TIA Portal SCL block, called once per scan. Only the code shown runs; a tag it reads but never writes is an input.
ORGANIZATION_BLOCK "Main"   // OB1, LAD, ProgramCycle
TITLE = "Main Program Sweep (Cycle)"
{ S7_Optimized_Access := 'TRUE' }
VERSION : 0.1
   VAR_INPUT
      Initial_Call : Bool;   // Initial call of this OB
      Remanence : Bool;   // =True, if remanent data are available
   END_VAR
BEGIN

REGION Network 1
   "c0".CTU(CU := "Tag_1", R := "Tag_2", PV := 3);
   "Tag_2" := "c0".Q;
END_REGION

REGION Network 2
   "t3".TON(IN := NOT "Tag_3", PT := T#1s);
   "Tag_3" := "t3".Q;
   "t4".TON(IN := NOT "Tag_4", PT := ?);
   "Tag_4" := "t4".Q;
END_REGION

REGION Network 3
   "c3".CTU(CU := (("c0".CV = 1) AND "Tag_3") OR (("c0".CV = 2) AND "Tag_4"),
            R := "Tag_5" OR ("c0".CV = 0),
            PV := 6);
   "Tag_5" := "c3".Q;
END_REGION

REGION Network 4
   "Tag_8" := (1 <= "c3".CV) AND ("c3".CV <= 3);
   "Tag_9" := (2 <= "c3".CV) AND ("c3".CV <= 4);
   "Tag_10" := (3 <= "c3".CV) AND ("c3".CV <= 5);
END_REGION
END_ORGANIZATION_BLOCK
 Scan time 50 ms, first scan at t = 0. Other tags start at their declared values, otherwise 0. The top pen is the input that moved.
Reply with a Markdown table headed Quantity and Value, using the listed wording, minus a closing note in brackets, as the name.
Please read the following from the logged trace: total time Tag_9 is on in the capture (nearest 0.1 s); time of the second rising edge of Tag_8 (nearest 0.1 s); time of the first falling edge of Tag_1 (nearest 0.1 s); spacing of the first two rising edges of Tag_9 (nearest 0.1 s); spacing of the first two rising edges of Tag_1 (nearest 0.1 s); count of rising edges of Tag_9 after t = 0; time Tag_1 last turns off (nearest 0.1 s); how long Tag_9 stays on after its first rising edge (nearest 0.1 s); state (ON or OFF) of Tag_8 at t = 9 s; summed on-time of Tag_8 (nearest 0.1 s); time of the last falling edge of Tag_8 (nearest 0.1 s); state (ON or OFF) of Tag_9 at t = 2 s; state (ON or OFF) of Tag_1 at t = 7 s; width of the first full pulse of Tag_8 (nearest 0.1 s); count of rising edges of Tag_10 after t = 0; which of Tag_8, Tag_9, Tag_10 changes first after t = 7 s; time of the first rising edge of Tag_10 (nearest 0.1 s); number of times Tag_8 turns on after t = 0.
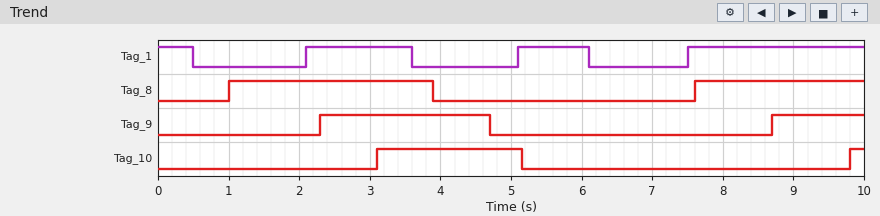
| Quantity | Value |
|---|---|
| total time Tag_9 is on in the capture | 3.7 s |
| time of the second rising edge of Tag_8 | 7.6 s |
| time of the first falling edge of Tag_1 | 0.5 s |
| spacing of the first two rising edges of Tag_9 | 6.4 s |
| spacing of the first two rising edges of Tag_1 | 3.0 s |
| count of rising edges of Tag_9 after t = 0 | 2 |
| time Tag_1 last turns off | 6.1 s |
| how long Tag_9 stays on after its first rising edge | 2.4 s |
| state (ON or OFF) of Tag_8 at t = 9 s | ON |
| summed on-time of Tag_8 | 5.3 s |
| time of the last falling edge of Tag_8 | 3.9 s |
| state (ON or OFF) of Tag_9 at t = 2 s | OFF |
| state (ON or OFF) of Tag_1 at t = 7 s | OFF |
| width of the first full pulse of Tag_8 | 2.9 s |
| count of rising edges of Tag_10 after t = 0 | 2 |
| which of Tag_8, Tag_9, Tag_10 changes first after t = 7 s | Tag_8 |
| time of the first rising edge of Tag_10 | 3.1 s |
| number of times Tag_8 turns on after t = 0 | 2 |
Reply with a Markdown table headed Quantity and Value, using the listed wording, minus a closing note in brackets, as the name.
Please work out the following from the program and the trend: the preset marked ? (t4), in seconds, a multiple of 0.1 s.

| Quantity | Value |
|---|---|
| the preset marked ? (t4), in seconds, a multiple of 0.1 s | 0.7 s |
